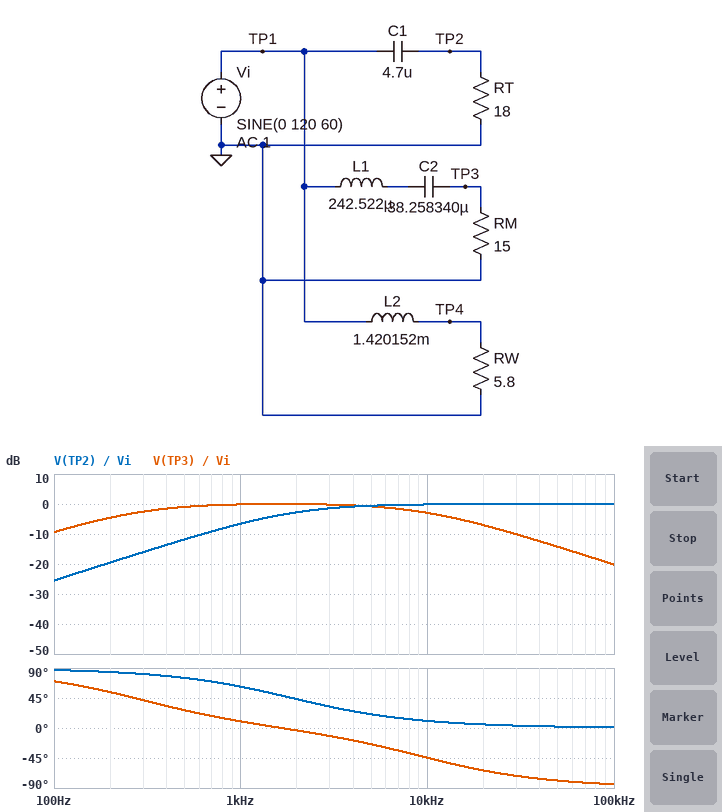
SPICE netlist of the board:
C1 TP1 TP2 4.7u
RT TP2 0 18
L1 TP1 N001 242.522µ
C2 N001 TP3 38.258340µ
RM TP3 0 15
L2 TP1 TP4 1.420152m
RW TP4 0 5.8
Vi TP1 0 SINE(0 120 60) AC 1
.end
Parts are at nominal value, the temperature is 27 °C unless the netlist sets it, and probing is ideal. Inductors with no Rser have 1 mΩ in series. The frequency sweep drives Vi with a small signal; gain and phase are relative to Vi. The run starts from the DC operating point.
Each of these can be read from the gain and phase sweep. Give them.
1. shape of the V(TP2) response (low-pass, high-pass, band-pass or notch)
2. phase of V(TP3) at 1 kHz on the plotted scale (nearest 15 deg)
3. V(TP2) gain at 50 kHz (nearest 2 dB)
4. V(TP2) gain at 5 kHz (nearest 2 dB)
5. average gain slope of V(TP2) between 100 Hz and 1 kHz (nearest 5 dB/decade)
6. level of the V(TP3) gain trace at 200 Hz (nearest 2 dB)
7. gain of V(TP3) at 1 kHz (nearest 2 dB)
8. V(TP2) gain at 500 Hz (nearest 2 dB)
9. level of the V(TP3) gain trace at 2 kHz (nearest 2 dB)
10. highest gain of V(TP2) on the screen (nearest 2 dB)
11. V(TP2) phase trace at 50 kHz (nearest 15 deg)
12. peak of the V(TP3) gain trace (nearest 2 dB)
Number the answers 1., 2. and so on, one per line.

1. high-pass
2. 15 deg
3. 0 dB
4. 0 dB
5. 20 dB/decade
6. -4 dB
7. 0 dB
8. -12 dB
9. 0 dB
10. 0 dB
11. 0 deg
12. 0 dB
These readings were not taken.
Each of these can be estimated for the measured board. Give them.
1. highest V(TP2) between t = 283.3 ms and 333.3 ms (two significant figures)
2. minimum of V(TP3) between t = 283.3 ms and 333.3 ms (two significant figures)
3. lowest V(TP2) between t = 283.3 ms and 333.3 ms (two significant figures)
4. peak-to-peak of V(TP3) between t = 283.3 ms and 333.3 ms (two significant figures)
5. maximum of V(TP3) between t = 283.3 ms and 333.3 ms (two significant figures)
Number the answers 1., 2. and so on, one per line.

1. 3.8 V
2. -25 V
3. -3.8 V
4. 51 V
5. 25 V
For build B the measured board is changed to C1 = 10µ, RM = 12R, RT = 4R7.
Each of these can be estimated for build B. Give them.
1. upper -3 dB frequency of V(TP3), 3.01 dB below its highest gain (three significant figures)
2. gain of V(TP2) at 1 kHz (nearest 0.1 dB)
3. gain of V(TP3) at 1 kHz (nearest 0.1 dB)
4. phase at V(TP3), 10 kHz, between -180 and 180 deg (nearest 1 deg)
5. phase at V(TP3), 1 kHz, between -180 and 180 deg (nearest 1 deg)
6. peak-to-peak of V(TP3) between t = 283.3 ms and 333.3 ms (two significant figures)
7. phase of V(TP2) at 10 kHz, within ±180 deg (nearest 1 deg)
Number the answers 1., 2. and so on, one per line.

1. 8.21 kHz
2. -11.0 dB
3. -0.2 dB
4. -51 deg
5. 12 deg
6. 41 V
7. 19 deg
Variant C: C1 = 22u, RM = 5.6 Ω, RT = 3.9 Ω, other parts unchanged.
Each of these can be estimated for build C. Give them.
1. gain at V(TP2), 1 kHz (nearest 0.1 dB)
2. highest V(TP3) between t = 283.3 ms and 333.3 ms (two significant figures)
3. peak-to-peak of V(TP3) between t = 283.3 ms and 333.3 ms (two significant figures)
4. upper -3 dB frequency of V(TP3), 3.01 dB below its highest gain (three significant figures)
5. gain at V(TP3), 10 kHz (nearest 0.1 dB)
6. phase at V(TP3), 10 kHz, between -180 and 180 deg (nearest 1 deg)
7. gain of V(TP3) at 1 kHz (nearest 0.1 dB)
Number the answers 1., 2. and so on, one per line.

1. -6.5 dB
2. 9.7 V
3. 19 V
4. 4.31 kHz
5. -9.0 dB
6. -69 deg
7. -0.9 dB
